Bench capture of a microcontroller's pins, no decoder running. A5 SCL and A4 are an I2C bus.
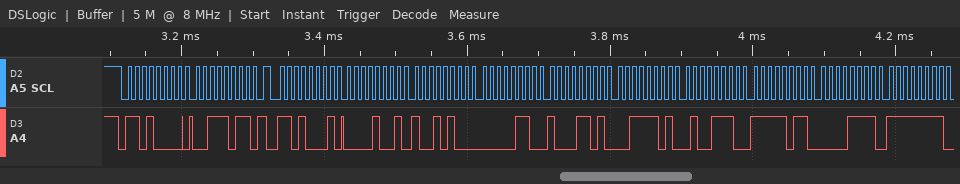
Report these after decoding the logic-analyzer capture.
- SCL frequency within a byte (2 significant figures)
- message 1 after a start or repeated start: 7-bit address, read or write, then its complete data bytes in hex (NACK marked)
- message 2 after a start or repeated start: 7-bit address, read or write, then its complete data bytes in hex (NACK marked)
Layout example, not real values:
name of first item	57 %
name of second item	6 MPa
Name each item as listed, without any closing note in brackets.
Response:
SCL frequency within a byte	100 kHz
message 1 after a start or repeated start: 7-bit address, read or write, then its complete data bytes in hex	0x68 write: 3B
message 2 after a start or repeated start: 7-bit address, read or write, then its complete data bytes in hex	0x68 read: 09 94 06 8D 3D 4E FB 0F FF
